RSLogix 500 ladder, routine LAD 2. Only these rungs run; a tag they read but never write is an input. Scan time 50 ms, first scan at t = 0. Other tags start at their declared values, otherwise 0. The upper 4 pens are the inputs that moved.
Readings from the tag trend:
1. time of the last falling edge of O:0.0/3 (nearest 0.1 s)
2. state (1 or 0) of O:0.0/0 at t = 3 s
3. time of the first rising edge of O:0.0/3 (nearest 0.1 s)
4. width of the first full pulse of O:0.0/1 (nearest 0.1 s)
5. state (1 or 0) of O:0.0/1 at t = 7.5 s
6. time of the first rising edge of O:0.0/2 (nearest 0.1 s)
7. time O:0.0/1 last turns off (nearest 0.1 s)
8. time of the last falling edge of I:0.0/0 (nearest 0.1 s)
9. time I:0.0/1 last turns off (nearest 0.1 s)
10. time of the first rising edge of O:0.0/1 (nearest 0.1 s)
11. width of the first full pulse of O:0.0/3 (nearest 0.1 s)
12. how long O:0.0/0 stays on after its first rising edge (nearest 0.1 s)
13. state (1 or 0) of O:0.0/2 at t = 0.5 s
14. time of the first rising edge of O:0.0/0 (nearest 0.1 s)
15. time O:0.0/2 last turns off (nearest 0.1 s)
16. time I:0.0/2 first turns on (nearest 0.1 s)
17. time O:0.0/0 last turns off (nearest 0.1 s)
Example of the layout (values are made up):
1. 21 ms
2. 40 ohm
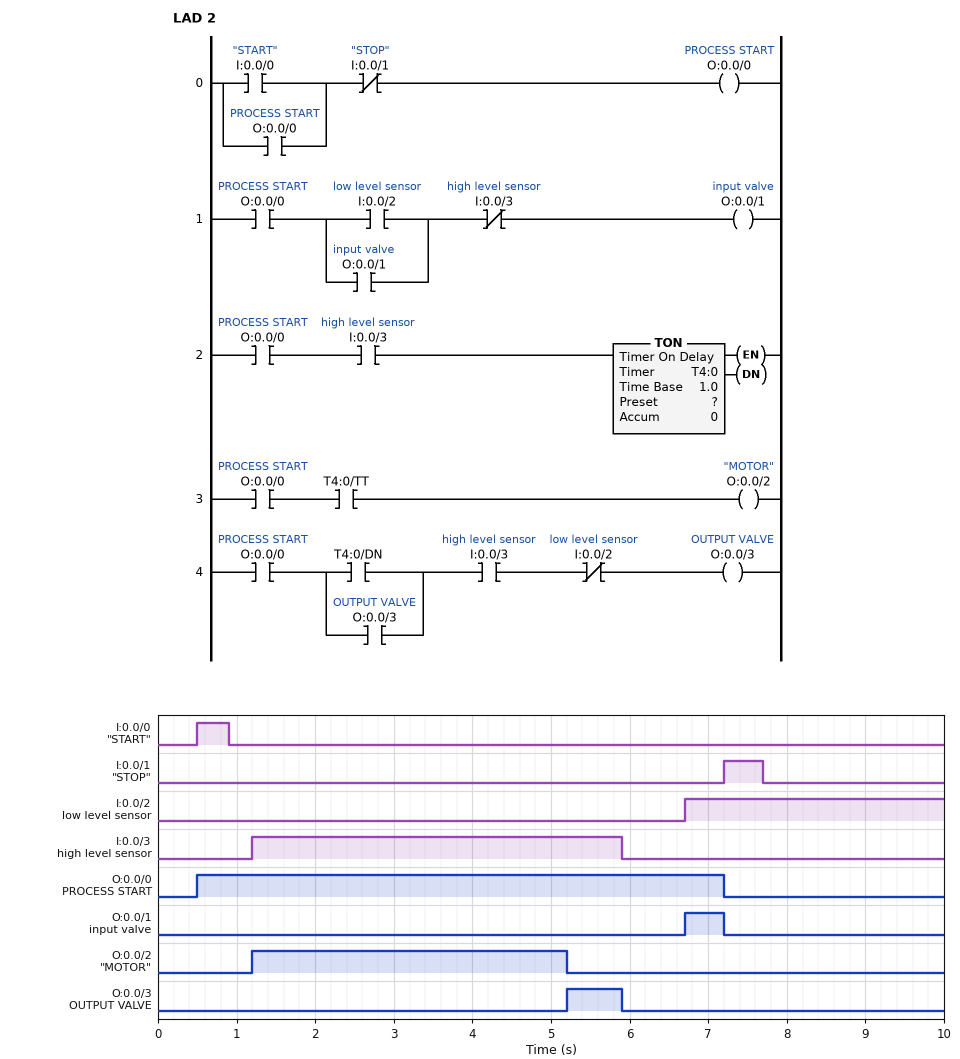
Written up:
1. 5.9 s
2. 1
3. 5.2 s
4. 0.5 s
5. 0
6. 1.2 s
7. 7.2 s
8. 0.9 s
9. 7.7 s
10. 6.7 s
11. 0.7 s
12. 6.7 s
13. 0
14. 0.5 s
15. 5.2 s
16. 6.7 s
17. 7.2 s
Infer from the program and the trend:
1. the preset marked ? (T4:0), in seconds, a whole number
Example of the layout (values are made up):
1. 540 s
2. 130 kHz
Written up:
1. 4 s
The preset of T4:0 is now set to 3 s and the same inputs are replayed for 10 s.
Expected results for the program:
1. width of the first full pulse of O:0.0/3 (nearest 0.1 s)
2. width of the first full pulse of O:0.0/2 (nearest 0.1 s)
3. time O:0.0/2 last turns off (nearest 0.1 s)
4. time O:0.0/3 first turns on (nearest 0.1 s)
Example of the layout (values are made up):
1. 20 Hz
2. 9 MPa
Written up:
1. 1.7 s
2. 3.0 s
3. 4.2 s
4. 4.2 s
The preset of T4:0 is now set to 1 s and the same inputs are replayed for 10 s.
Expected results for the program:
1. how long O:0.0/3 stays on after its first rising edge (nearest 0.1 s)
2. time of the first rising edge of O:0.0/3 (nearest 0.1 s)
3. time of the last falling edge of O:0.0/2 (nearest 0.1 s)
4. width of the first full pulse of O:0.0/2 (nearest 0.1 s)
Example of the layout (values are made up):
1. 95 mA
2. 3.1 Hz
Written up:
1. 3.7 s
2. 2.2 s
3. 2.2 s
4. 1.0 s
